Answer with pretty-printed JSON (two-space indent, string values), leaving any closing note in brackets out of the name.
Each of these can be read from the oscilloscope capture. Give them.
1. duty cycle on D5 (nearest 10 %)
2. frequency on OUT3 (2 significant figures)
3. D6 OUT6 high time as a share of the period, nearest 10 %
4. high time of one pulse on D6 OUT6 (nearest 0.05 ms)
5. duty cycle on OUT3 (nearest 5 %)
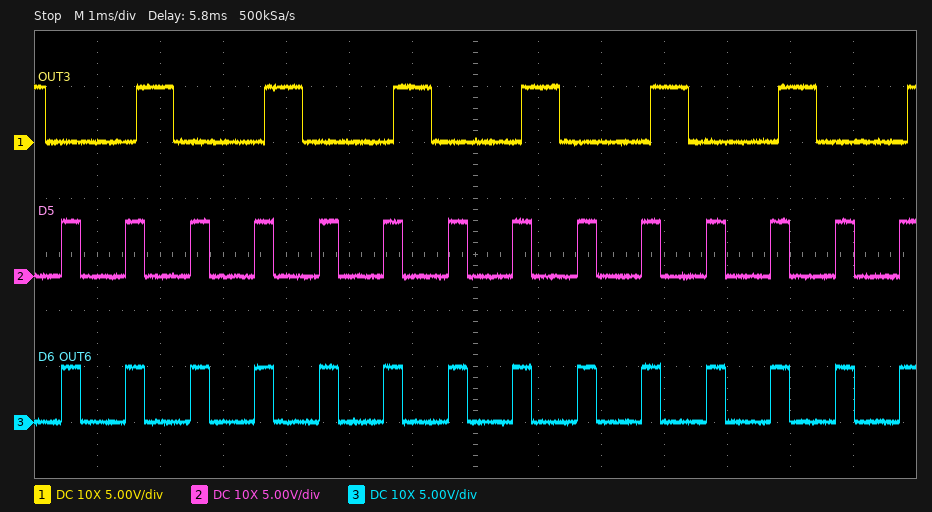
{
  "duty cycle on D5": "30 %",
  "frequency on OUT3": "490 Hz",
  "D6 OUT6 high time as a share of the period, nearest 10 %": "30 %",
  "high time of one pulse on D6 OUT6": "0.30 ms",
  "duty cycle on OUT3": "30 %"
}
